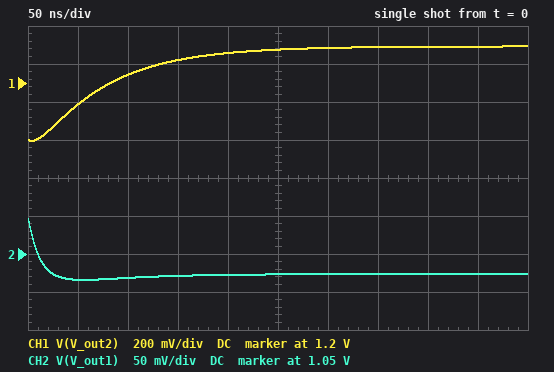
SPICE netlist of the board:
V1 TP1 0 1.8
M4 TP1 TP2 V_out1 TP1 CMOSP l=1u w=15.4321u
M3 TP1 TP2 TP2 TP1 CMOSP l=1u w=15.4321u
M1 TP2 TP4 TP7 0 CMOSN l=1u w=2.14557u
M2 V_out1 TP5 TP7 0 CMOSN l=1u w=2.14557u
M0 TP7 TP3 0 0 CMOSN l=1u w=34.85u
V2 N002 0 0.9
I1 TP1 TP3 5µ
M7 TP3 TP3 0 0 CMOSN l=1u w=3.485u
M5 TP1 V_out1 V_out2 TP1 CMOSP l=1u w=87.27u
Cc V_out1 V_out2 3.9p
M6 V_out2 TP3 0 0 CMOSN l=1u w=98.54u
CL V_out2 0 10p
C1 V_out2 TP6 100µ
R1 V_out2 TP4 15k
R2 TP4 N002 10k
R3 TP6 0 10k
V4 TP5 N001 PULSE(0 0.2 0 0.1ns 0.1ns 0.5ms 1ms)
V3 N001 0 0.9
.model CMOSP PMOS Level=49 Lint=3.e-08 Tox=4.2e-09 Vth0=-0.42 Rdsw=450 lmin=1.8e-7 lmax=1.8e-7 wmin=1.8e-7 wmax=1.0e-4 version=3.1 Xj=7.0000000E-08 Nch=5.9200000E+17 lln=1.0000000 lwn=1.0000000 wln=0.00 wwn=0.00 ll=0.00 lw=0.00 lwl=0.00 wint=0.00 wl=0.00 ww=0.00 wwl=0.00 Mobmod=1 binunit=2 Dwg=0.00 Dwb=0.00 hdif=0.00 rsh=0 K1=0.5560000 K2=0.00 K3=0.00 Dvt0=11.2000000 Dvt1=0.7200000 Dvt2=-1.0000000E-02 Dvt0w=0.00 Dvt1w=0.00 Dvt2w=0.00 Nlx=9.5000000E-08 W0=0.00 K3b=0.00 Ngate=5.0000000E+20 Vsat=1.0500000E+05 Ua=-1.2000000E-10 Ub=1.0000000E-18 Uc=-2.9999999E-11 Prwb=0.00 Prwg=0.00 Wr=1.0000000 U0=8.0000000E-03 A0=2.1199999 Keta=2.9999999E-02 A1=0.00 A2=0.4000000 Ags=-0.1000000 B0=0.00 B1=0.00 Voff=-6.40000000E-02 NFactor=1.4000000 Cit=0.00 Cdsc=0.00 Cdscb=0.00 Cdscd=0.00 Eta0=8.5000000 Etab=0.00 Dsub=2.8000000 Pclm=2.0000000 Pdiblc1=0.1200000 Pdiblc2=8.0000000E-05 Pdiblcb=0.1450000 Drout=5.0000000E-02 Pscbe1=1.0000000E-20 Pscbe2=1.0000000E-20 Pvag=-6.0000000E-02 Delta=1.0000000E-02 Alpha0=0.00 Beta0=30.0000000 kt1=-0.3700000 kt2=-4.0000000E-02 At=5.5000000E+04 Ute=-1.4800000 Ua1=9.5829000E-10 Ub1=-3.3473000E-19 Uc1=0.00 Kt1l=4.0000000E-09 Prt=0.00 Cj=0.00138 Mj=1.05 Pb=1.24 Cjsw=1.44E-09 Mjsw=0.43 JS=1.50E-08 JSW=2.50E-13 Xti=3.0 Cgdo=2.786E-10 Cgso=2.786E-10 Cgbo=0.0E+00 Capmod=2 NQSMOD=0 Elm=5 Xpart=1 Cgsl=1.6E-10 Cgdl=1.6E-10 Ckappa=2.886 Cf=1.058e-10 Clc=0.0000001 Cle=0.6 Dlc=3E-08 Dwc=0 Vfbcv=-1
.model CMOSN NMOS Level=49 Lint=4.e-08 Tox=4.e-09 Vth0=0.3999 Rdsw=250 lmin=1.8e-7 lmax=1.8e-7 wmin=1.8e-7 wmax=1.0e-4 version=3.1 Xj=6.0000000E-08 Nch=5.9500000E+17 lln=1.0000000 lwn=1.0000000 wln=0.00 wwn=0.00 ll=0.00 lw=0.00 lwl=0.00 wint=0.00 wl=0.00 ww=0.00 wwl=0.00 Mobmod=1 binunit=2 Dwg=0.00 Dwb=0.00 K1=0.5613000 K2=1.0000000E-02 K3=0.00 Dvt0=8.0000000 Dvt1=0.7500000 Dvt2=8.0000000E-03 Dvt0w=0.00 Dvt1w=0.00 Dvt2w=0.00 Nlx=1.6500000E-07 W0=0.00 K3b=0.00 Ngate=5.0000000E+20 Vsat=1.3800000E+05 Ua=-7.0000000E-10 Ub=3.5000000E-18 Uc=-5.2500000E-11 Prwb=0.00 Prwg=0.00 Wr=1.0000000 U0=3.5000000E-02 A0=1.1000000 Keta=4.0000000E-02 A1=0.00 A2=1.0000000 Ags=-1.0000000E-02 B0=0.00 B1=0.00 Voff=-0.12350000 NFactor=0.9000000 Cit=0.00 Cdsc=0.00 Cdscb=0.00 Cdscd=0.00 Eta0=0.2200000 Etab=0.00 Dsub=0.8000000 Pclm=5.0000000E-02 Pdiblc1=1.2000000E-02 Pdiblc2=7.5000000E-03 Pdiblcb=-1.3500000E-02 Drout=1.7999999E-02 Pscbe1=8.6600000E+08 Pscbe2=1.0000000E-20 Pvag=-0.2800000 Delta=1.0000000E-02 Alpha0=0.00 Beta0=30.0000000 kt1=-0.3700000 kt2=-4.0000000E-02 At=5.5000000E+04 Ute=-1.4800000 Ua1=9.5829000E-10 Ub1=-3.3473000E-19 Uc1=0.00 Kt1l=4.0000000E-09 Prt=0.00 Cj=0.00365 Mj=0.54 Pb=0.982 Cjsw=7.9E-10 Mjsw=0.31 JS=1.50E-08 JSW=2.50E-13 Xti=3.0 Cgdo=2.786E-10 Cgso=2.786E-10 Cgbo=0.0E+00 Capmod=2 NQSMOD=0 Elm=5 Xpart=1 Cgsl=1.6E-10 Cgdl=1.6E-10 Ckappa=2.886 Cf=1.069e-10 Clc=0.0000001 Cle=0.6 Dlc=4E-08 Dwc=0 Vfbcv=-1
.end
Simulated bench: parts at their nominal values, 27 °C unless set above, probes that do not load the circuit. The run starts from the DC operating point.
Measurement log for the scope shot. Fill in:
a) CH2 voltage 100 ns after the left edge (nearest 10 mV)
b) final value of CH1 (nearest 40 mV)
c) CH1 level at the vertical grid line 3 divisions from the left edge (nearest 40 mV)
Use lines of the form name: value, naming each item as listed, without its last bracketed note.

CH2 voltage 100 ns after the left edge: 1.02 V
final value of CH1: 1.40 V
CH1 level at the vertical grid line 3 divisions from the left edge: 1.32 V
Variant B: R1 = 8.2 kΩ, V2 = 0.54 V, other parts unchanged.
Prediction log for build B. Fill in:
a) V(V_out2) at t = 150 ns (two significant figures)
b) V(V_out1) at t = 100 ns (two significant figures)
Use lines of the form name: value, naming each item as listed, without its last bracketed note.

V(V_out2) at t = 150 ns: 1.5 V
V(V_out1) at t = 100 ns: 990 mV
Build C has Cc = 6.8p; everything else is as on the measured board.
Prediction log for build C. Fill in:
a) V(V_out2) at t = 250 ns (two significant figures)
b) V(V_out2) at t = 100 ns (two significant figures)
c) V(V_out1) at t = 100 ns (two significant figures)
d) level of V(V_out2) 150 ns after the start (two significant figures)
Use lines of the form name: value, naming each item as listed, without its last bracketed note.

V(V_out2) at t = 250 ns: 1.3 V
V(V_out2) at t = 100 ns: 1.1 V
V(V_out1) at t = 100 ns: 1.0 V
level of V(V_out2) 150 ns after the start: 1.2 V
